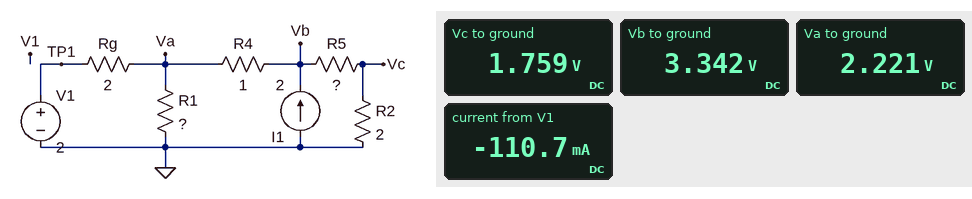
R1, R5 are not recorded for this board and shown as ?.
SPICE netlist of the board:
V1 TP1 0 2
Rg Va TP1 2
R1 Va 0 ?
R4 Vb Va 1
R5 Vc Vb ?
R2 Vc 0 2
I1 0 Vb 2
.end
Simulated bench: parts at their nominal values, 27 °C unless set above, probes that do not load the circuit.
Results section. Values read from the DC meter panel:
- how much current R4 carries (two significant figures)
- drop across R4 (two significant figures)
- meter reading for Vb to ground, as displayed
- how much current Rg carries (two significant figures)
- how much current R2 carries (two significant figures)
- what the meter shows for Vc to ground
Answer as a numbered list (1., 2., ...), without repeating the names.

1. 1.1 A
2. 1.1 V
3. 3.342 V
4. 110 mA
5. 880 mA
6. 1.759 V
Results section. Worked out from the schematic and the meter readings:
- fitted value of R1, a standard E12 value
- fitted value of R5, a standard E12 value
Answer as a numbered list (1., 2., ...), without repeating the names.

1. 2.2 Ω
2. 1.8 Ω
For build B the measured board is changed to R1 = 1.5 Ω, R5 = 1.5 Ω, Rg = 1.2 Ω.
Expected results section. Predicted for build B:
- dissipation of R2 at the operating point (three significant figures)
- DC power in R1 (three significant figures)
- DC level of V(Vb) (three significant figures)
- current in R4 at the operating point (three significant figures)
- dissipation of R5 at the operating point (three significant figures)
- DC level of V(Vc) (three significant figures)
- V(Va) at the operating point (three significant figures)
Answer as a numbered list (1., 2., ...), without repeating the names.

1. 1.48 W
2. 2.33 W
3. 3.01 V
4. 1.14 A
5. 1.11 W
6. 1.72 V
7. 1.87 V
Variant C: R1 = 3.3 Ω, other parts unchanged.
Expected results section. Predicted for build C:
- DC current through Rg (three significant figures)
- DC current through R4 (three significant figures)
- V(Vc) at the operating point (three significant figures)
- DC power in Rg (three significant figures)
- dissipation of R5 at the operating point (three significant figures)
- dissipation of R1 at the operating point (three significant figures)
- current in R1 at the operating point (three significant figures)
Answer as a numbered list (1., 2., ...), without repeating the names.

1. 277 mA
2. 1.05 A
3. 1.90 V
4. 154 mW
5. 1.62 W
6. 1.98 W
7. 774 mA
